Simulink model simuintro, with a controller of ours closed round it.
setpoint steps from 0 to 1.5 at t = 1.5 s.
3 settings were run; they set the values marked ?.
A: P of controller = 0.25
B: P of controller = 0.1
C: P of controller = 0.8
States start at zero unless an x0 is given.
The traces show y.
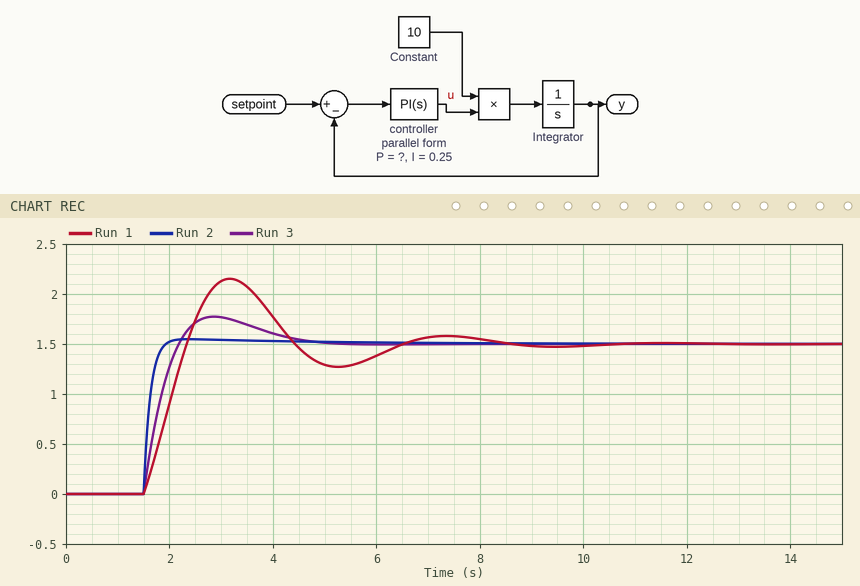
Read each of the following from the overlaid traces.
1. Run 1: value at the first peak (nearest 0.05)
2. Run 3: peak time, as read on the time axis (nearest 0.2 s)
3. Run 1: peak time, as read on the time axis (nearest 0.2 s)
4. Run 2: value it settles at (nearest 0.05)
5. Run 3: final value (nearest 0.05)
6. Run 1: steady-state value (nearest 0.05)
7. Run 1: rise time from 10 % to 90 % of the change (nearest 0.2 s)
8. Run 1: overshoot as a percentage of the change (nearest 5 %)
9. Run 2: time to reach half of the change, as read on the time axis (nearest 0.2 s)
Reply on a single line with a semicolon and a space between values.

2.15; 2.8 s; 3.2 s; 1.50; 1.50; 1.50; 0.6 s; 45 %; 1.6 s
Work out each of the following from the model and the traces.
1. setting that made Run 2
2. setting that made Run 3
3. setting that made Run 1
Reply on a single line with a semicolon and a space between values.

C; A; B
